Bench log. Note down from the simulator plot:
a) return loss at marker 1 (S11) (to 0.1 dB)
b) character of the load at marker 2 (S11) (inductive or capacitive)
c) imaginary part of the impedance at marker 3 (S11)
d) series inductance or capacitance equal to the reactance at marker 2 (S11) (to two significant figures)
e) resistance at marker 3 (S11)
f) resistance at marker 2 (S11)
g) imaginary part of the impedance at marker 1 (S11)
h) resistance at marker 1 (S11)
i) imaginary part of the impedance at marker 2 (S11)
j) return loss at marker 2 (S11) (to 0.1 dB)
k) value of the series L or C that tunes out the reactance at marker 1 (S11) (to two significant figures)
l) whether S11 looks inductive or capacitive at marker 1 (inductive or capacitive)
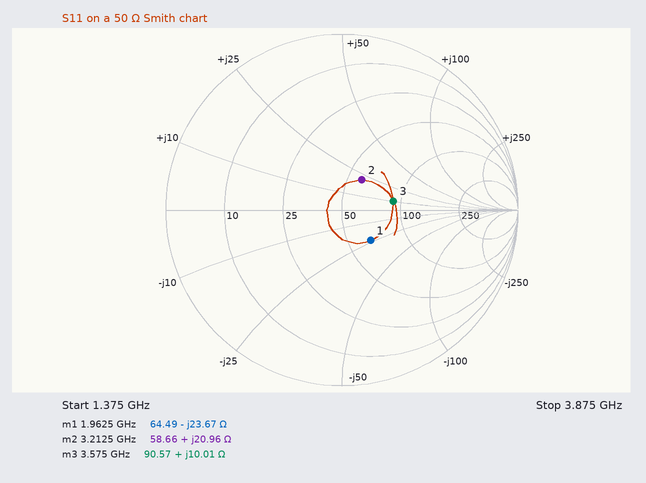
12.5 dB
inductive
+10.01 Ω
1.0 nH
90.57 Ω
58.66 Ω
-23.67 Ω
64.49 Ω
+20.96 Ω
13.8 dB
1.9 nH
capacitive
